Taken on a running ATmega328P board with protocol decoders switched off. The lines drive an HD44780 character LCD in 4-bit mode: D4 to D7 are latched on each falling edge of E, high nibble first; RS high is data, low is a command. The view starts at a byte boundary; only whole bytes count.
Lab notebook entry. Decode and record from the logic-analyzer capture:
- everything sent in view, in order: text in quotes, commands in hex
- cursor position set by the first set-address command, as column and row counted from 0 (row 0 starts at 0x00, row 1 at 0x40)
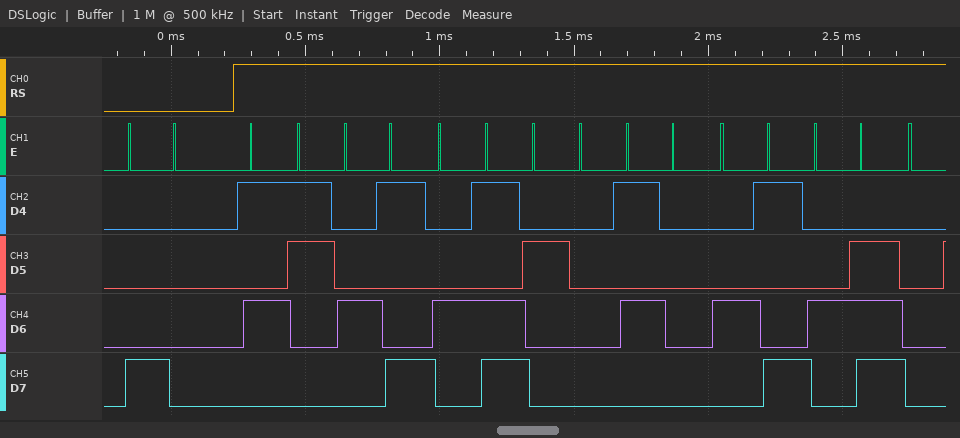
0x80 "SIM PIN"
column 0, row 0
